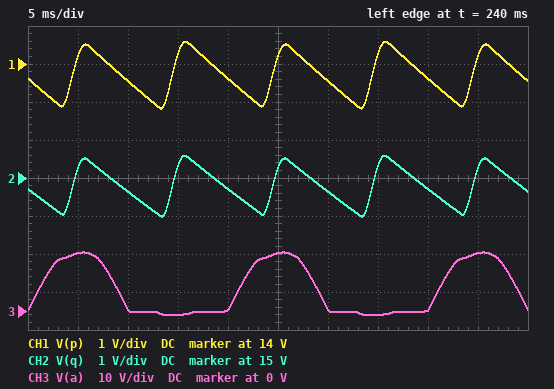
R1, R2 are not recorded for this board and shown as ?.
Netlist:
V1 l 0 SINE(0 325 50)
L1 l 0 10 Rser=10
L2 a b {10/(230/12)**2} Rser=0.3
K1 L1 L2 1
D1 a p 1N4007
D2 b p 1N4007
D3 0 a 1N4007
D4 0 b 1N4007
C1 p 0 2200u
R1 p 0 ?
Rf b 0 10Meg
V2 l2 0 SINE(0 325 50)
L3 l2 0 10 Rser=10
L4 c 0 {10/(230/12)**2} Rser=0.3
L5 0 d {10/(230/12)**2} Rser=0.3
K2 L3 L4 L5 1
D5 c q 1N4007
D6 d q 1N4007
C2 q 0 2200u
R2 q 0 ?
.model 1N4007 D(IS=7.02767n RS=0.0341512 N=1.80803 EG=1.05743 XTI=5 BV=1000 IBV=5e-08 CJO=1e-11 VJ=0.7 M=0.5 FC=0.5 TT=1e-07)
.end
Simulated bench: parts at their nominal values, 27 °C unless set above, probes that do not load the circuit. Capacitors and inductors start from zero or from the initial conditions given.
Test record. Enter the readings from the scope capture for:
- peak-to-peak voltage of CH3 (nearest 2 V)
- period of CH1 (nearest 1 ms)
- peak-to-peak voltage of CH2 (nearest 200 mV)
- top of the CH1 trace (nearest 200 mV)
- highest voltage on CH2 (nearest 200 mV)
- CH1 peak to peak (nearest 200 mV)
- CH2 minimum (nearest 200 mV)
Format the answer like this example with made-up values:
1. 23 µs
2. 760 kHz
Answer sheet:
1. 16 V
2. 10 ms
3. 1.6 V
4. 14.6 V
5. 15.6 V
6. 1.8 V
7. 14.0 V
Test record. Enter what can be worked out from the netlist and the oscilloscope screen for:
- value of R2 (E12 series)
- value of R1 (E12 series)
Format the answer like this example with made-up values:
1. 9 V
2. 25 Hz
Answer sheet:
1. 33 Ω
2. 27 Ω
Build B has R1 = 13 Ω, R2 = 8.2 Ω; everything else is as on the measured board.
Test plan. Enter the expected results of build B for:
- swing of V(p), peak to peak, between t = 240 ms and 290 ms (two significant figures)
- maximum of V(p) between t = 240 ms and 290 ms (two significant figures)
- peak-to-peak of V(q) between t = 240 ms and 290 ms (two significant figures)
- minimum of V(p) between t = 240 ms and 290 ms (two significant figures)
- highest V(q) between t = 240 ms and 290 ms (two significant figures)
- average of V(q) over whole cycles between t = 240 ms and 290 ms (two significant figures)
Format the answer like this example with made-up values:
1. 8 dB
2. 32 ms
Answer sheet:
1. 3.1 V
2. 14 V
3. 4.5 V
4. 11 V
5. 15 V
6. 13 V
